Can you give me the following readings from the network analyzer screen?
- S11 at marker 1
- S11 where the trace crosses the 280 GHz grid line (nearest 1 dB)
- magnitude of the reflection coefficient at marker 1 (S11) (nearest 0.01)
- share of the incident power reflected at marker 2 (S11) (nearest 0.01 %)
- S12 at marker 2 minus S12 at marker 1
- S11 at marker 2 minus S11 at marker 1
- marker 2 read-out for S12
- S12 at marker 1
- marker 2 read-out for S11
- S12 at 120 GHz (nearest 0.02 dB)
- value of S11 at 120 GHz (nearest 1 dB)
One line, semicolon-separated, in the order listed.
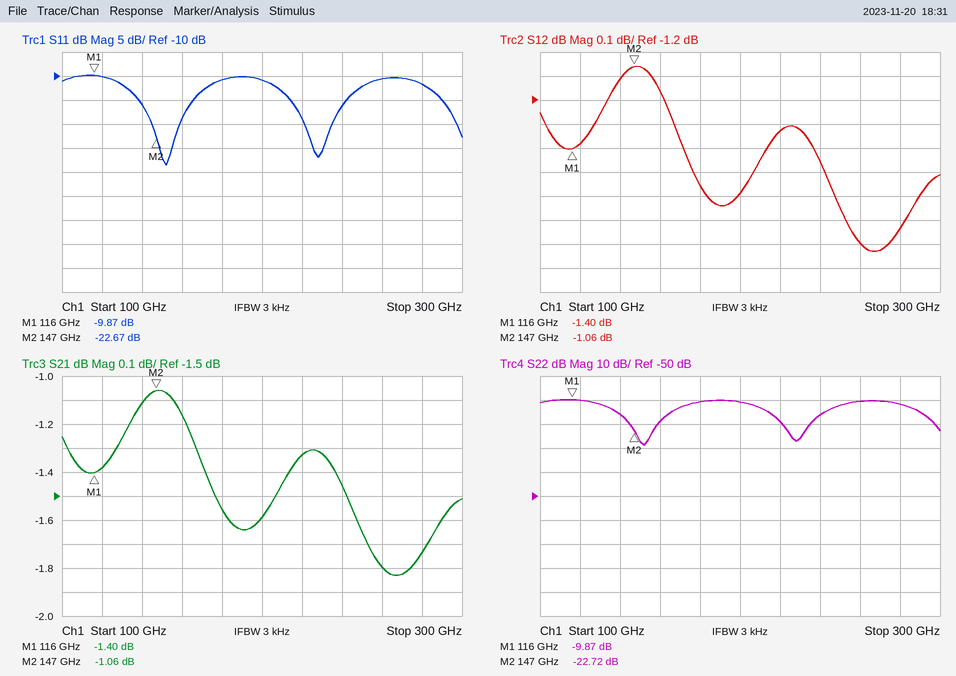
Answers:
-9.87 dB; -12 dB; 0.32; 0.54 %; 0.34 dB; -12.80 dB; -1.06 dB; -1.40 dB; -22.67 dB; -1.38 dB; -10 dB
